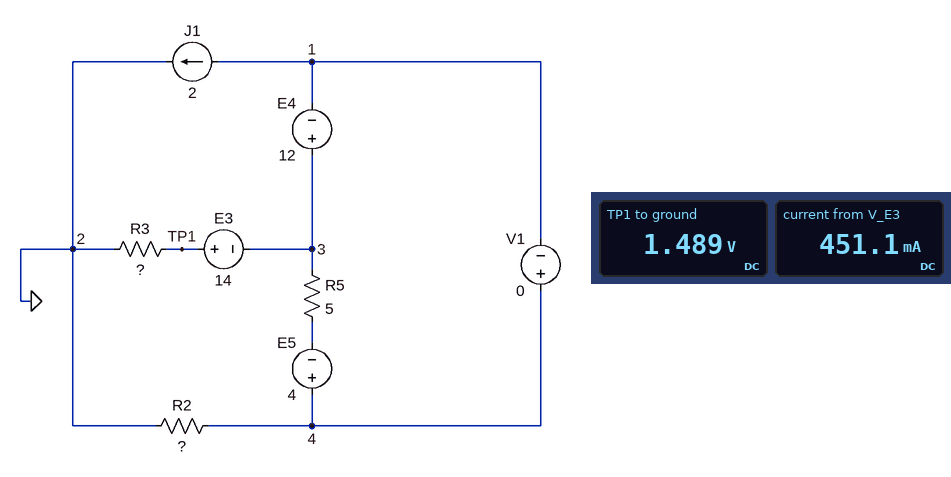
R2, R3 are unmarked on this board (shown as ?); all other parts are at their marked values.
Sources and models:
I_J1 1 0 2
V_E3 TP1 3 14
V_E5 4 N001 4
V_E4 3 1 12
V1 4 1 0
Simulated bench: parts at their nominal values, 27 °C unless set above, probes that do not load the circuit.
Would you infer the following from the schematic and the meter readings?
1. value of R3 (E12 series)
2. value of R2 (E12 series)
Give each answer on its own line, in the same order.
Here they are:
3.3 Ω
10 Ω
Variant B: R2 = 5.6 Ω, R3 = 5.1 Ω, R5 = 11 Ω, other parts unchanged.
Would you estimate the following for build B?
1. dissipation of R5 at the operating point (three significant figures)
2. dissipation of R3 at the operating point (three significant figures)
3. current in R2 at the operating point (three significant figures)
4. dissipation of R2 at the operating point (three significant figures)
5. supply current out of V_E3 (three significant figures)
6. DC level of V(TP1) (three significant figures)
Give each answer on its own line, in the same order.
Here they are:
23.3 W
9.76 W
3.38 A
64.1 W
1.38 A
7.05 V
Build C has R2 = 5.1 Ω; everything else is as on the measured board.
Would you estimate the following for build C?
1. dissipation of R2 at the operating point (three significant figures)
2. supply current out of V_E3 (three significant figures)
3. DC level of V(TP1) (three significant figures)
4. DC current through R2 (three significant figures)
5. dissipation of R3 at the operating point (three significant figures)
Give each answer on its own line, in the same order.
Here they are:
76.8 W
1.88 A
6.21 V
3.88 A
11.7 W
